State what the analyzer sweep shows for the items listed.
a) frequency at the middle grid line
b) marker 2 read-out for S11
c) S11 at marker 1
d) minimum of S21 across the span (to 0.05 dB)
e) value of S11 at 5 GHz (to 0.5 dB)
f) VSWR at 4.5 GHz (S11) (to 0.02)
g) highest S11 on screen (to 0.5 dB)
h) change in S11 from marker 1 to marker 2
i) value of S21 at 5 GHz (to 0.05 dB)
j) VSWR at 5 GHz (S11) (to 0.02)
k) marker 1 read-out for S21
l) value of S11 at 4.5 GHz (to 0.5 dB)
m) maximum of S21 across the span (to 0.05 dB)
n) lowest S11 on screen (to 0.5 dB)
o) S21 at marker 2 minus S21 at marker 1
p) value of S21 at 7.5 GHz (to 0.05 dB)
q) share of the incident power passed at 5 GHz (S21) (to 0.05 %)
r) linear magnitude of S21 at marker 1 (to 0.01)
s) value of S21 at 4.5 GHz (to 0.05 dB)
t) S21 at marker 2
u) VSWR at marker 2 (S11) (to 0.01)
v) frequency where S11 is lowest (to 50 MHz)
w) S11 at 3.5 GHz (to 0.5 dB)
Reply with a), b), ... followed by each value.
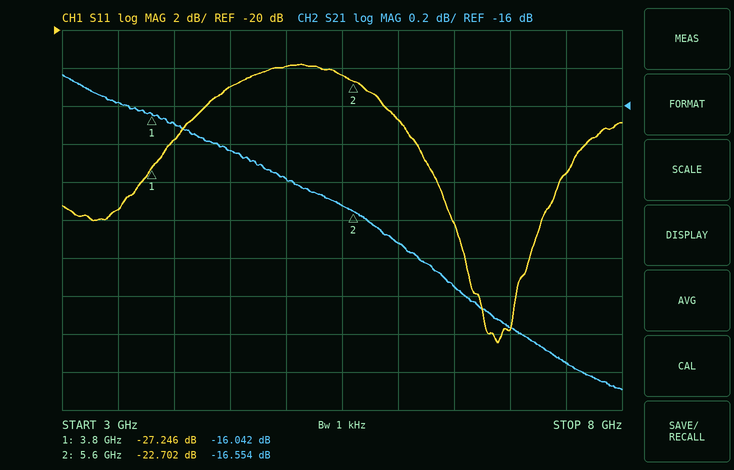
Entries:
a) 5.5 GHz
b) -22.702 dB
c) -27.246 dB
d) -17.50 dB
e) -22.0 dB
f) 1.16
g) -22.0 dB
h) 4.544 dB
i) -16.40 dB
j) 1.18
k) -16.042 dB
l) -23.0 dB
m) -15.85 dB
n) -36.5 dB
o) -0.512 dB
p) -17.35 dB
q) 2.30 %
r) 0.16
s) -16.25 dB
t) -16.554 dB
u) 1.16
v) 6.90 GHz
w) -29.5 dB
